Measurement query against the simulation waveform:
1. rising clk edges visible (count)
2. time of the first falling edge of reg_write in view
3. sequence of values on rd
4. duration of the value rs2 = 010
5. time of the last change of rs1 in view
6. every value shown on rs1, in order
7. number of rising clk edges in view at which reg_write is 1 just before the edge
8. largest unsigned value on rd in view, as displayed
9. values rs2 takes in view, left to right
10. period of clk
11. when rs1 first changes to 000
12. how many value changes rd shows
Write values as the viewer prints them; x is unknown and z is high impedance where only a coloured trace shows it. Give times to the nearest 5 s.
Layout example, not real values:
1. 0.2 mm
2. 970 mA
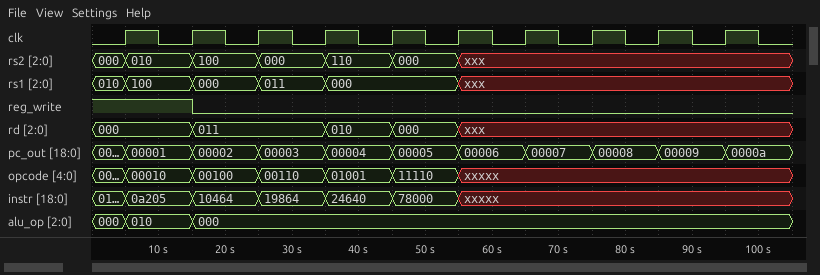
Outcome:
1. 10
2. 15 s
3. 000, 011, 010, 000, xxx
4. 10 s
5. 55 s
6. 010, 100, 000, 011, 000, xxx
7. 2
8. 011
9. 000, 010, 100, 000, 110, 000, xxx
10. 10 s
11. 15 s
12. 4
